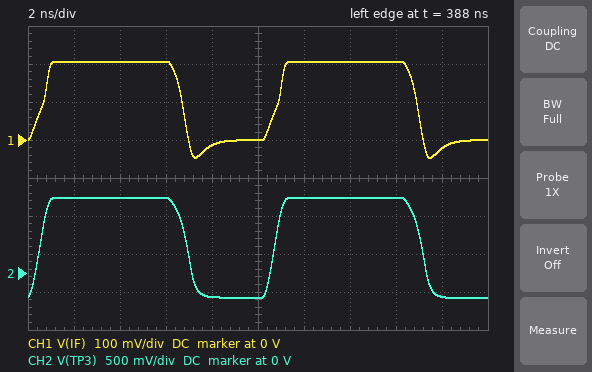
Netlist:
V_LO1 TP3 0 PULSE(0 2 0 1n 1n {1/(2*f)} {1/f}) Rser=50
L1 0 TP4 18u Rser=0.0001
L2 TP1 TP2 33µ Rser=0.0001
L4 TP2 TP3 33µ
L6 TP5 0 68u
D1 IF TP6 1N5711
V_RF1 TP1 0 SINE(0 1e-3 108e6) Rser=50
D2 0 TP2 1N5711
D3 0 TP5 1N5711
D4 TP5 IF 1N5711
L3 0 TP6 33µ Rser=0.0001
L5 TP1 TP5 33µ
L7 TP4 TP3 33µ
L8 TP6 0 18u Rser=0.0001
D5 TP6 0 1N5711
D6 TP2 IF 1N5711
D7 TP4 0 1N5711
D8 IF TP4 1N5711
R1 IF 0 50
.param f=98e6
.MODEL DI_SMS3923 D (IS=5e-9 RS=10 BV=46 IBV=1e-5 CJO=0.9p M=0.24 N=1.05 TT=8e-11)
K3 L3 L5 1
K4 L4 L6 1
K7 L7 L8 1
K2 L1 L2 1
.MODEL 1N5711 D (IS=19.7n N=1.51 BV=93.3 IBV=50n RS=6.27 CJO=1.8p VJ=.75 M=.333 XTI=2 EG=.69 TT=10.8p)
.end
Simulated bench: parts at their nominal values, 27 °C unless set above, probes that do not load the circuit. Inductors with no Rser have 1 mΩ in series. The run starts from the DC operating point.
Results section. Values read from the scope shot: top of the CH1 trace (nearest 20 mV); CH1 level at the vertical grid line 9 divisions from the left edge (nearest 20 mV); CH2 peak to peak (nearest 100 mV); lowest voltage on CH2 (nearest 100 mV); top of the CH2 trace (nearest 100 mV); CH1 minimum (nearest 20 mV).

200 mV
-20 mV
1.3 V
-300 mV
1.0 V
-40 mV
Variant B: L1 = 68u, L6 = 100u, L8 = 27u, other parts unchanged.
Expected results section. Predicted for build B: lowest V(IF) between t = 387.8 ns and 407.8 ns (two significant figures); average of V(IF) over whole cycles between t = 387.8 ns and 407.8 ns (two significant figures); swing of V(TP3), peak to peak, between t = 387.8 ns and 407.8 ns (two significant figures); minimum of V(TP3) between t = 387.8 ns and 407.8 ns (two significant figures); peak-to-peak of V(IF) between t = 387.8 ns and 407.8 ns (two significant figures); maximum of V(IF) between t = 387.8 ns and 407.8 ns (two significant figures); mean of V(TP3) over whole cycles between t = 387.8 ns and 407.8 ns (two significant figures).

-49 mV
180 mV
750 mV
-82 mV
370 mV
320 mV
390 mV
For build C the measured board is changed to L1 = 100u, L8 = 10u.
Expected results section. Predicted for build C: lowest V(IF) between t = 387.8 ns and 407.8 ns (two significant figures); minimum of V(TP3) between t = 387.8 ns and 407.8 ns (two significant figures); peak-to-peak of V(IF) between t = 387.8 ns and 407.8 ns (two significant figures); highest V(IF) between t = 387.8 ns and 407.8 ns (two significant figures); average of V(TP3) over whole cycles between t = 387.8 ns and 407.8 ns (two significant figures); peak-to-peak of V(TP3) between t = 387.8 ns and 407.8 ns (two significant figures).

-97 mV
-150 mV
390 mV
290 mV
210 mV
550 mV
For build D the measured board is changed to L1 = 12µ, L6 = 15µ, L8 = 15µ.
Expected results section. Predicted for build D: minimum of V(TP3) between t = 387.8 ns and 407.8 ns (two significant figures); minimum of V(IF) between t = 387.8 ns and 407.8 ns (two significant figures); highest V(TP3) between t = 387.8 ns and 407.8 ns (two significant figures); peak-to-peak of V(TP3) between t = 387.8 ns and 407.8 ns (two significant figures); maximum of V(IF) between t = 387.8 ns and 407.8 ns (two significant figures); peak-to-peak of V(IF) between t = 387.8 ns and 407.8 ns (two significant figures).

-470 mV
-110 mV
1.1 V
1.6 V
160 mV
270 mV
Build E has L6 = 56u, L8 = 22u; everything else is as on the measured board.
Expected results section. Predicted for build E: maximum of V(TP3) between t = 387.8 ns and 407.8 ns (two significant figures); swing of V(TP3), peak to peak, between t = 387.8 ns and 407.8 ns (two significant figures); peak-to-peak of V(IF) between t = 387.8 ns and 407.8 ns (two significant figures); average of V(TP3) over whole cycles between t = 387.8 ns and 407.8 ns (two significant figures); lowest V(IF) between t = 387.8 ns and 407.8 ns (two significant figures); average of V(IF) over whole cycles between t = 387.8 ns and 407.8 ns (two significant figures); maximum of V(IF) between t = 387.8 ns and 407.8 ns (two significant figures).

1.0 V
1.4 V
150 mV
510 mV
-24 mV
75 mV
130 mV
